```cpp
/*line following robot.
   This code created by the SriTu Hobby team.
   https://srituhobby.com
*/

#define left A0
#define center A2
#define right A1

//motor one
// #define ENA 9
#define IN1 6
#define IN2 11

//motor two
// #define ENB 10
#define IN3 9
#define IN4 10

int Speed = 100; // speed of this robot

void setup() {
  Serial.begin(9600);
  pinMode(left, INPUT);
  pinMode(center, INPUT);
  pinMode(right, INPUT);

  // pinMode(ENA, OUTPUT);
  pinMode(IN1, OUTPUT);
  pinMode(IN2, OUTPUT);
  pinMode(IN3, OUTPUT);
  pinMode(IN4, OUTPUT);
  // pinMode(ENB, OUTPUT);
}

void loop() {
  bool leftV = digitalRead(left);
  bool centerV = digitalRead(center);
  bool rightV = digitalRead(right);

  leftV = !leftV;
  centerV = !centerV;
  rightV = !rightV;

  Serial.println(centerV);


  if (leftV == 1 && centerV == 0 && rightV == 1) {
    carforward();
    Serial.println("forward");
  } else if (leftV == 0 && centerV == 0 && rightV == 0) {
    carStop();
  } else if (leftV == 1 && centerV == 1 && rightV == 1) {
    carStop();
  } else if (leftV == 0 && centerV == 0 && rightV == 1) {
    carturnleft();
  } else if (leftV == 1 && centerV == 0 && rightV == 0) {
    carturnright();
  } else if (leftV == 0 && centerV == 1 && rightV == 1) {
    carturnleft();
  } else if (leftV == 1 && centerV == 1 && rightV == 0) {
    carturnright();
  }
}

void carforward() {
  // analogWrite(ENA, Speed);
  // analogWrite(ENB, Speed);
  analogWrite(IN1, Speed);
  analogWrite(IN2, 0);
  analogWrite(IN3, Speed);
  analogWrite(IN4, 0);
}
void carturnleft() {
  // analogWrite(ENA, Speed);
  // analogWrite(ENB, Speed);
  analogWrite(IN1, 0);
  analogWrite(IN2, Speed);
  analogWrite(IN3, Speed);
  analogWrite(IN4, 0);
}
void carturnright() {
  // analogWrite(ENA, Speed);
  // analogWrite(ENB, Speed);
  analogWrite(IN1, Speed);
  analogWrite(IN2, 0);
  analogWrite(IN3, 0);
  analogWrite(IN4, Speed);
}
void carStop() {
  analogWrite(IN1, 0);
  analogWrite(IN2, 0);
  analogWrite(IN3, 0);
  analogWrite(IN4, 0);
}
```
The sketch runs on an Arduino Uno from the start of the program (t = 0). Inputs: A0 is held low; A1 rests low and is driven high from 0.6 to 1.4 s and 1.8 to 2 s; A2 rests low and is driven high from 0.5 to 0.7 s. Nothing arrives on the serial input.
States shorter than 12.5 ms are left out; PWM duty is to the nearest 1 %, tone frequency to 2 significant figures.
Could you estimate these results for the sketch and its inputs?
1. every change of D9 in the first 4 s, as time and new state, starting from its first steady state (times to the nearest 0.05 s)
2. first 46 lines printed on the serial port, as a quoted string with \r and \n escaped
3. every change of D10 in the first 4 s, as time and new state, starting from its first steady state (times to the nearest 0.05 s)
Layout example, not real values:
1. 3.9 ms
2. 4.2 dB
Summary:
1. 0 s low; 0.5 s PWM 39 %; 0.6 s low
2. "1\r\n1\r\n1\r\n1\r\n1\r\n1\r\n1\r\n1\r\n1\r\n1\r\n1\r\n1\r\n1\r\n1\r\n1\r\n1\r\n1\r\n1\r\n1\r\n1\r\n1\r\n1\r\n1\r\n1\r\n1\r\n1\r\n1\r\n1\r\n1\r\n1\r\n1\r\n1\r\n1\r\n1\r\n1\r\n1\r\n1\r\n1\r\n1\r\n1\r\n1\r\n1\r\n1\r\n1\r\n1\r\n1\r\n"
3. 0 s low; 0.6 s PWM 39 %; 1.4 s low; 1.8 s PWM 39 %; 2 s low
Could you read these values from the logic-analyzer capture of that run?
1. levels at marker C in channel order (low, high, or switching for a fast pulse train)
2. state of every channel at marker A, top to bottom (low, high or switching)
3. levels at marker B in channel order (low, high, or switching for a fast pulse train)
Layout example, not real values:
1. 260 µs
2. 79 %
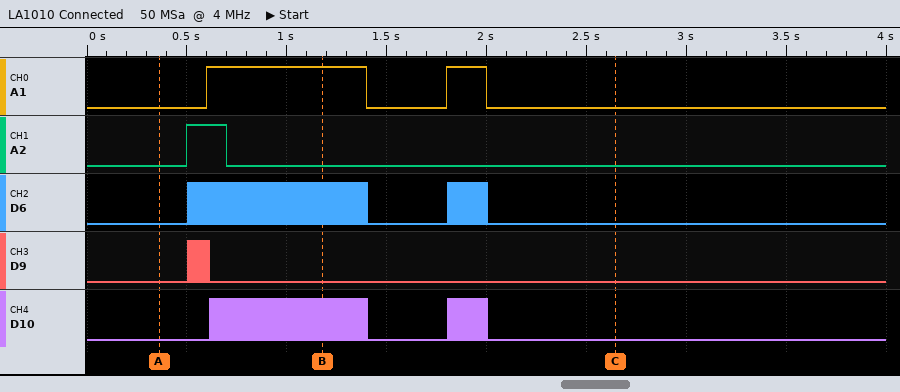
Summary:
1. A1 low, A2 low, D6 low, D9 low, D10 low
2. A1 low, A2 low, D6 low, D9 low, D10 low
3. A1 high, A2 low, D6 switching, D9 low, D10 switching
